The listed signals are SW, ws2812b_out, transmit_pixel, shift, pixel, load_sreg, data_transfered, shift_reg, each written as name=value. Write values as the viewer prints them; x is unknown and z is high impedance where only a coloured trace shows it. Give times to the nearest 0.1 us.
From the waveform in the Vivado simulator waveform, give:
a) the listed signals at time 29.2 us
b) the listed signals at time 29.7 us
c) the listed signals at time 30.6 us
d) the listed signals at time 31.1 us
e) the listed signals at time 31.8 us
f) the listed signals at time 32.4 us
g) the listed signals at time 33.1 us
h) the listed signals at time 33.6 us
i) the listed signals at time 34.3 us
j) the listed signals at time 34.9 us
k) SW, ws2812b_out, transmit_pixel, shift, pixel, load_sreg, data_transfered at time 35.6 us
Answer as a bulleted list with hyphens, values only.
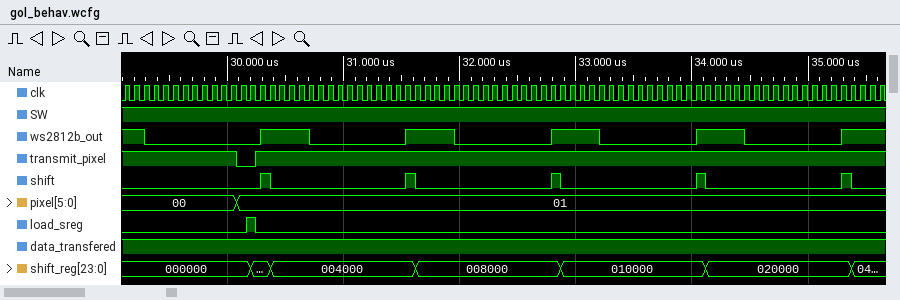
- SW=1, ws2812b_out=1, transmit_pixel=1, shift=0, pixel=00, load_sreg=0, data_transfered=1, shift_reg=000000
- SW=1, ws2812b_out=0, transmit_pixel=1, shift=0, pixel=00, load_sreg=0, data_transfered=1, shift_reg=000000
- SW=1, ws2812b_out=1, transmit_pixel=1, shift=0, pixel=01, load_sreg=0, data_transfered=1, shift_reg=004000
- SW=1, ws2812b_out=0, transmit_pixel=1, shift=0, pixel=01, load_sreg=0, data_transfered=1, shift_reg=004000
- SW=1, ws2812b_out=1, transmit_pixel=1, shift=0, pixel=01, load_sreg=0, data_transfered=1, shift_reg=008000
- SW=1, ws2812b_out=0, transmit_pixel=1, shift=0, pixel=01, load_sreg=0, data_transfered=1, shift_reg=008000
- SW=1, ws2812b_out=1, transmit_pixel=1, shift=0, pixel=01, load_sreg=0, data_transfered=1, shift_reg=010000
- SW=1, ws2812b_out=0, transmit_pixel=1, shift=0, pixel=01, load_sreg=0, data_transfered=1, shift_reg=010000
- SW=1, ws2812b_out=1, transmit_pixel=1, shift=0, pixel=01, load_sreg=0, data_transfered=1, shift_reg=020000
- SW=1, ws2812b_out=0, transmit_pixel=1, shift=0, pixel=01, load_sreg=0, data_transfered=1, shift_reg=020000
- SW=1, ws2812b_out=1, transmit_pixel=1, shift=0, pixel=01, load_sreg=0, data_transfered=1
